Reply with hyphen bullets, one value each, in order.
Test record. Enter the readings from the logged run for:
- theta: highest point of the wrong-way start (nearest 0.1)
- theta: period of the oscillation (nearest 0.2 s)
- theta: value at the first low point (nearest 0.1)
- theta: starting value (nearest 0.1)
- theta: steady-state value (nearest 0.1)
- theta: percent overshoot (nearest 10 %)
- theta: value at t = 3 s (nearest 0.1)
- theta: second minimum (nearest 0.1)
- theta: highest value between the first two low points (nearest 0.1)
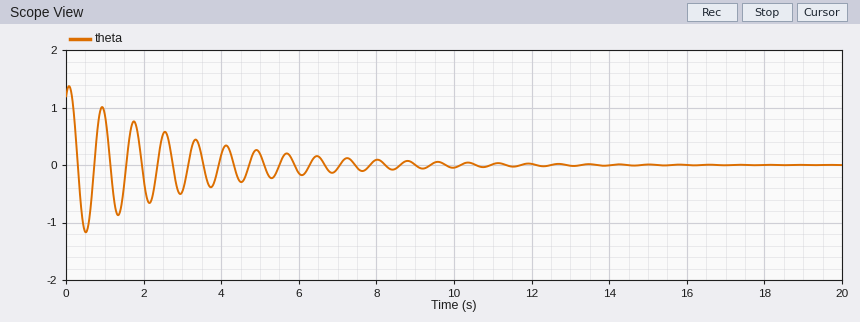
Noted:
- 1.4
- 0.8 s
- -1.2
- 1.2
- 0.0
- 100 %
- -0.5
- -0.9
- 1.0
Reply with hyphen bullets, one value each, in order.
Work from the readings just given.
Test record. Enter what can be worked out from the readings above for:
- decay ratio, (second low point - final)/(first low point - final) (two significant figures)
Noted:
- 0.75
